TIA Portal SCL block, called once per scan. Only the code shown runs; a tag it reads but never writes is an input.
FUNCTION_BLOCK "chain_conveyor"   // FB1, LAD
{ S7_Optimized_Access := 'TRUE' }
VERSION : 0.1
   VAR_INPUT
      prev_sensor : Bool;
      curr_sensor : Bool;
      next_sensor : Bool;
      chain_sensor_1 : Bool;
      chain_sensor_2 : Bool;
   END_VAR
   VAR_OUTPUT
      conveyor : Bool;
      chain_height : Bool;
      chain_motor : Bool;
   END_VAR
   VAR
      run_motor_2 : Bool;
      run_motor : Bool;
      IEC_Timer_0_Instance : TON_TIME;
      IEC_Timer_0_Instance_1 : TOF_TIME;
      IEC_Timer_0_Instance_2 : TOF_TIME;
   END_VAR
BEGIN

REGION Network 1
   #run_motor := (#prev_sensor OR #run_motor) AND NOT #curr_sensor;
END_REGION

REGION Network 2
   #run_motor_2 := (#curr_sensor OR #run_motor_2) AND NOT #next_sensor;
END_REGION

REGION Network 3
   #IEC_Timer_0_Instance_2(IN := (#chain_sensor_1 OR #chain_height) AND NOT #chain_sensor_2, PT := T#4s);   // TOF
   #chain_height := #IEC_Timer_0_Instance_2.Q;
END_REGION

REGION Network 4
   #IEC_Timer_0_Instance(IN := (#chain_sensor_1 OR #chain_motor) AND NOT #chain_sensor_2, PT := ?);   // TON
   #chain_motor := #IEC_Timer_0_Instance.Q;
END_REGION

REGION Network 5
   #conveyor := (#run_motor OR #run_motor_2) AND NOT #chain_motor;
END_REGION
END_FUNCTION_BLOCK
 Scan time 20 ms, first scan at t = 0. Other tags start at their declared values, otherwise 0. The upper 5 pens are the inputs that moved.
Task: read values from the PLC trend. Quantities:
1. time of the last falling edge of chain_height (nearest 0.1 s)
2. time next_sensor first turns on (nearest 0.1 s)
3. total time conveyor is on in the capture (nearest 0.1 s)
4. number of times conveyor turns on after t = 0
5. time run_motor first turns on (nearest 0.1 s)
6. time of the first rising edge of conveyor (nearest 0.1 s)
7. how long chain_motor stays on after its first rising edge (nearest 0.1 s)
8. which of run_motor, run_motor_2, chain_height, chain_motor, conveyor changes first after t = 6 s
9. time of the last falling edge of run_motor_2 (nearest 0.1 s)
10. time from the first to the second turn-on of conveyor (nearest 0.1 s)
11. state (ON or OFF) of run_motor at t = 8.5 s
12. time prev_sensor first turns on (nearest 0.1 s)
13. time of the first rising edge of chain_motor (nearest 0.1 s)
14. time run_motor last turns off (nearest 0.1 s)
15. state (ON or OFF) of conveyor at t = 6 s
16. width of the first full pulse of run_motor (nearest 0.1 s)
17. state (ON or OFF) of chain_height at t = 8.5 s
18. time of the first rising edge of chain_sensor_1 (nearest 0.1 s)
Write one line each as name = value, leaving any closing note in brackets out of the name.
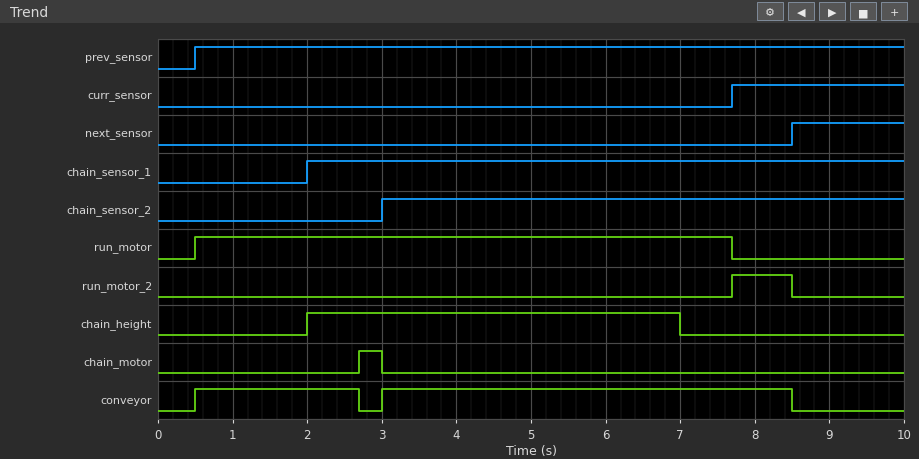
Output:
time of the last falling edge of chain_height = 7.0 s
time next_sensor first turns on = 8.5 s
total time conveyor is on in the capture = 7.7 s
number of times conveyor turns on after t = 0 = 2
time run_motor first turns on = 0.5 s
time of the first rising edge of conveyor = 0.5 s
how long chain_motor stays on after its first rising edge = 0.3 s
which of run_motor, run_motor_2, chain_height, chain_motor, conveyor changes first after t = 6 s = chain_height
time of the last falling edge of run_motor_2 = 8.5 s
time from the first to the second turn-on of conveyor = 2.5 s
state (ON or OFF) of run_motor at t = 8.5 s = OFF
time prev_sensor first turns on = 0.5 s
time of the first rising edge of chain_motor = 2.7 s
time run_motor last turns off = 7.7 s
state (ON or OFF) of conveyor at t = 6 s = ON
width of the first full pulse of run_motor = 7.2 s
state (ON or OFF) of chain_height at t = 8.5 s = OFF
time of the first rising edge of chain_sensor_1 = 2.0 s
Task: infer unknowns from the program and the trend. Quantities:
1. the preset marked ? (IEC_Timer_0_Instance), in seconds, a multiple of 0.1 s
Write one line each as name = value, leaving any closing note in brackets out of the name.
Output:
the preset marked ? (IEC_Timer_0_Instance), in seconds, a multiple of 0.1 s = 0.7 s
